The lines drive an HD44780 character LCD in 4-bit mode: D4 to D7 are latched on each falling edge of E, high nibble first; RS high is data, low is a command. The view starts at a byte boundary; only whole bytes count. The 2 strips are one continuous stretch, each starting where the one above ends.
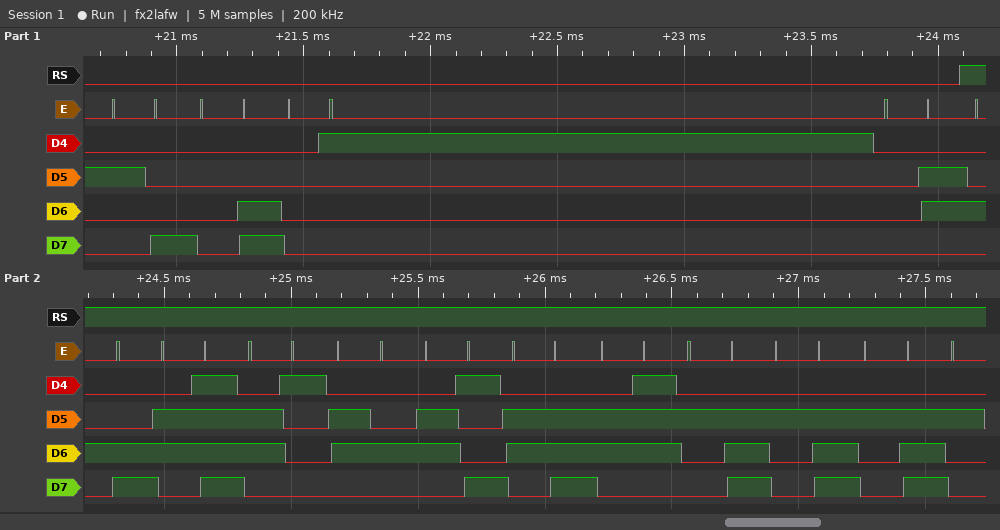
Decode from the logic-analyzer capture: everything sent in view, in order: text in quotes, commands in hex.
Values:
0x28 0x0C 0x01 0x06 "Loading..."
